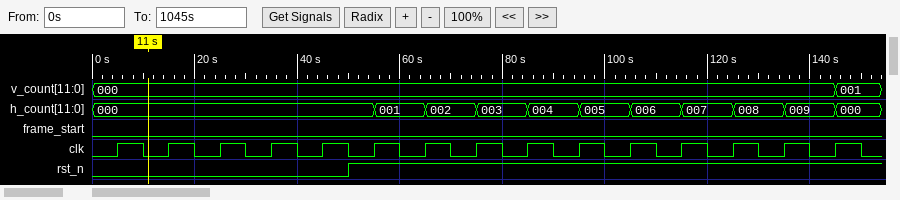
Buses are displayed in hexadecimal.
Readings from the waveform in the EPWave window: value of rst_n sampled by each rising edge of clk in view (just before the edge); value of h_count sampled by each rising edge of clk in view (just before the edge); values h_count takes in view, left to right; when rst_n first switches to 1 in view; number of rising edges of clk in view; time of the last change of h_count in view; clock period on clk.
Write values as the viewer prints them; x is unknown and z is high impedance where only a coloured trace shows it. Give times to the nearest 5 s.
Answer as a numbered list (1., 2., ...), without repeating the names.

1. 0 0 0 0 0 1 1 1 1 1 1 1 1 1 1
2. 000, 000, 000, 000, 000, 000, 001, 002, 003, 004, 005, 006, 007, 008, 009
3. 000, 001, 002, 003, 004, 005, 006, 007, 008, 009, 000
4. 50 s
5. 15
6. 145 s
7. 10 s
